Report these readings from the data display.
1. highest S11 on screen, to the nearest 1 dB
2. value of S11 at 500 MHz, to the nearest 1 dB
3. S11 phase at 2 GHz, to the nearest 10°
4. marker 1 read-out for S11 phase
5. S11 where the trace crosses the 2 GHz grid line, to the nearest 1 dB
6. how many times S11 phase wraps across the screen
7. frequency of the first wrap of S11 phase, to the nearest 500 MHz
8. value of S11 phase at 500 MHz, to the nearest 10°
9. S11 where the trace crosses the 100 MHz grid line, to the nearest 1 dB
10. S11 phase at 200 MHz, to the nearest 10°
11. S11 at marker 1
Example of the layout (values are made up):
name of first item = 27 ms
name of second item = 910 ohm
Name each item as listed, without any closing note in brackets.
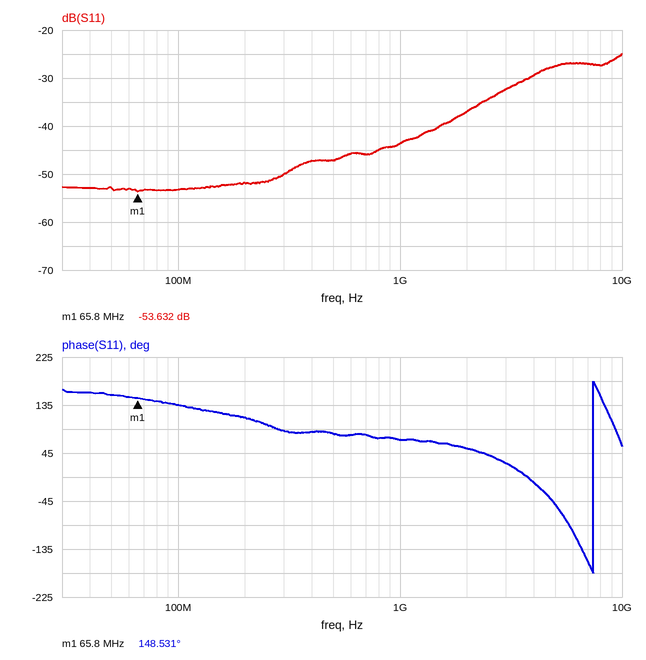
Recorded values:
highest S11 on screen, to the nearest 1 dB = -25 dB
value of S11 at 500 MHz, to the nearest 1 dB = -47 dB
S11 phase at 2 GHz, to the nearest 10° = 50°
marker 1 read-out for S11 phase = 148.531°
S11 where the trace crosses the 2 GHz grid line, to the nearest 1 dB = -37 dB
how many times S11 phase wraps across the screen = 1
frequency of the first wrap of S11 phase, to the nearest 500 MHz = 7.5 GHz
value of S11 phase at 500 MHz, to the nearest 10° = 80°
S11 where the trace crosses the 100 MHz grid line, to the nearest 1 dB = -53 dB
S11 phase at 200 MHz, to the nearest 10° = 110°
S11 at marker 1 = -53.632 dB
